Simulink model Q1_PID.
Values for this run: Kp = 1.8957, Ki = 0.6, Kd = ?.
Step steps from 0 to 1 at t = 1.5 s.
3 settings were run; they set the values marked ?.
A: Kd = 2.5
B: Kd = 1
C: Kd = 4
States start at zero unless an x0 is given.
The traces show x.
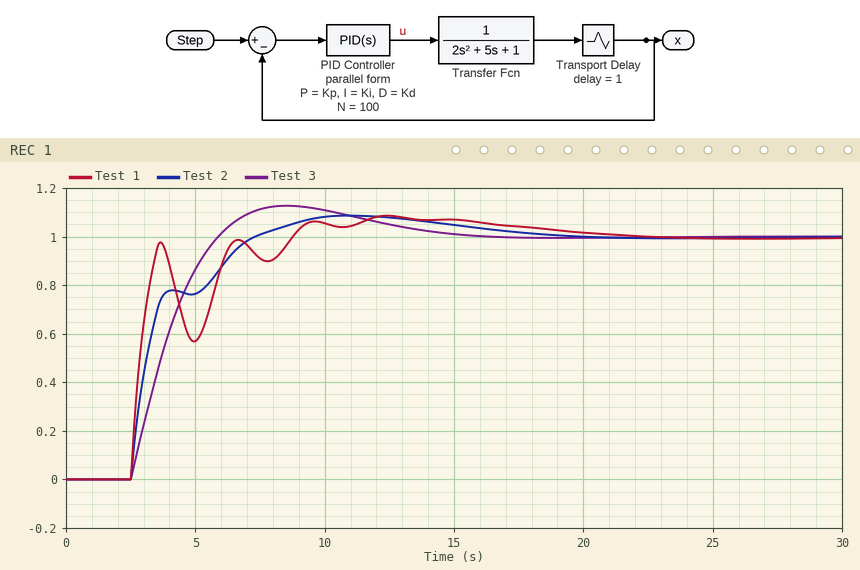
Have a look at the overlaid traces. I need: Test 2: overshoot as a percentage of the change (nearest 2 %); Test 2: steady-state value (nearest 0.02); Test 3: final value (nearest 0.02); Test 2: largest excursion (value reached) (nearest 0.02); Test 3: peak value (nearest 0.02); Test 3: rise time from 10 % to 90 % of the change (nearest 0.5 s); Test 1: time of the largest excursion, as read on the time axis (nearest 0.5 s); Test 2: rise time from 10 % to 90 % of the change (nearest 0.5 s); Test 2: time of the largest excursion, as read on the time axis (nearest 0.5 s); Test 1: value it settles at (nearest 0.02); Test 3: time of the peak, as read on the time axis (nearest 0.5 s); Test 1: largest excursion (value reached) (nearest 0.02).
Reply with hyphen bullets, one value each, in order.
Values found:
- 8 %
- 1.00
- 1.00
- 1.08
- 1.12
- 2.5 s
- 12.5 s
- 3.5 s
- 11.0 s
- 1.00
- 8.5 s
- 1.08
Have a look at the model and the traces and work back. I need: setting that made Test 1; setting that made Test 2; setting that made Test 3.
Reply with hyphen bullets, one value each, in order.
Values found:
- C
- A
- B
